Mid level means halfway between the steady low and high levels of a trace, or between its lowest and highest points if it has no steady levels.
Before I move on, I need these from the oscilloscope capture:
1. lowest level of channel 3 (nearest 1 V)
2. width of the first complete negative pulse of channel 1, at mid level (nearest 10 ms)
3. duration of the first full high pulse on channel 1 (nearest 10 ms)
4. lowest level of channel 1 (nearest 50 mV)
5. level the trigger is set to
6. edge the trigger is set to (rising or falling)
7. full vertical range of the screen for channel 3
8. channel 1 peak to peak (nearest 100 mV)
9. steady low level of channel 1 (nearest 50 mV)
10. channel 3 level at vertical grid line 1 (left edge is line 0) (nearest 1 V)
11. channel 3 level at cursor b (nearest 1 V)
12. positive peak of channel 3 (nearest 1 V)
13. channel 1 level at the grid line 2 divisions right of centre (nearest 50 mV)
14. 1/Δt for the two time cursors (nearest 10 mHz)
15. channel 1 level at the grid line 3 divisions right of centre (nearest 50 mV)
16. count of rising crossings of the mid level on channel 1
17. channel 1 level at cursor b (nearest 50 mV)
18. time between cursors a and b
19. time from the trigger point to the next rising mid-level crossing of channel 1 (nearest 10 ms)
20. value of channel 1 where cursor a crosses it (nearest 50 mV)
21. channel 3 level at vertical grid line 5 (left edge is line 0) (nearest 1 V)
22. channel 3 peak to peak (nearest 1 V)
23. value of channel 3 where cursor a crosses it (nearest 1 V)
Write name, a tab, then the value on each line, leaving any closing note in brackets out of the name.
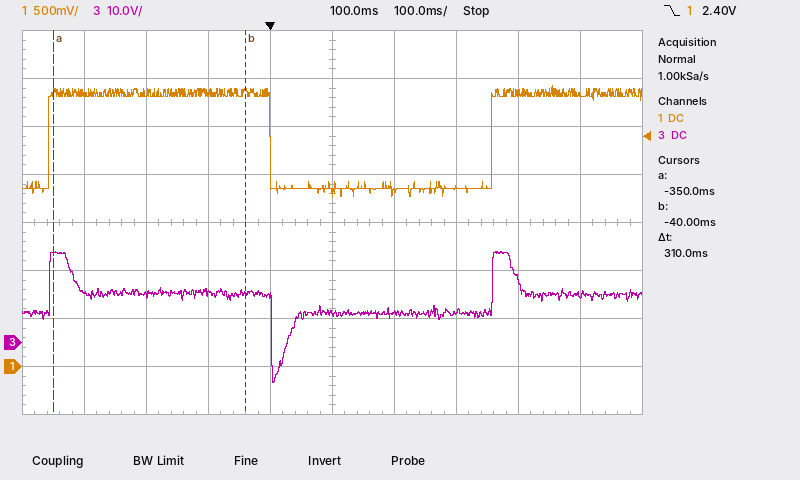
lowest level of channel 3	-8 V
width of the first complete negative pulse of channel 1, at mid level	360 ms
duration of the first full high pulse on channel 1	360 ms
lowest level of channel 1	1.75 V
level the trigger is set to	2.40 V
edge the trigger is set to	falling
full vertical range of the screen for channel 3	80 V
channel 1 peak to peak	1.20 V
steady low level of channel 1	1.85 V
channel 3 level at vertical grid line 1 (left edge is line 0)	10 V
channel 3 level at cursor b	10 V
positive peak of channel 3	19 V
channel 1 level at the grid line 2 divisions right of centre	1.85 V
1/Δt for the two time cursors	3.23 Hz
channel 1 level at the grid line 3 divisions right of centre	2.85 V
count of rising crossings of the mid level on channel 1	2
channel 1 level at cursor b	2.85 V
time between cursors a and b	310 ms
time from the trigger point to the next rising mid-level crossing of channel 1	360 ms
value of channel 1 where cursor a crosses it	2.85 V
channel 3 level at vertical grid line 5 (left edge is line 0)	6 V
channel 3 peak to peak	27 V
value of channel 3 where cursor a crosses it	18 V
